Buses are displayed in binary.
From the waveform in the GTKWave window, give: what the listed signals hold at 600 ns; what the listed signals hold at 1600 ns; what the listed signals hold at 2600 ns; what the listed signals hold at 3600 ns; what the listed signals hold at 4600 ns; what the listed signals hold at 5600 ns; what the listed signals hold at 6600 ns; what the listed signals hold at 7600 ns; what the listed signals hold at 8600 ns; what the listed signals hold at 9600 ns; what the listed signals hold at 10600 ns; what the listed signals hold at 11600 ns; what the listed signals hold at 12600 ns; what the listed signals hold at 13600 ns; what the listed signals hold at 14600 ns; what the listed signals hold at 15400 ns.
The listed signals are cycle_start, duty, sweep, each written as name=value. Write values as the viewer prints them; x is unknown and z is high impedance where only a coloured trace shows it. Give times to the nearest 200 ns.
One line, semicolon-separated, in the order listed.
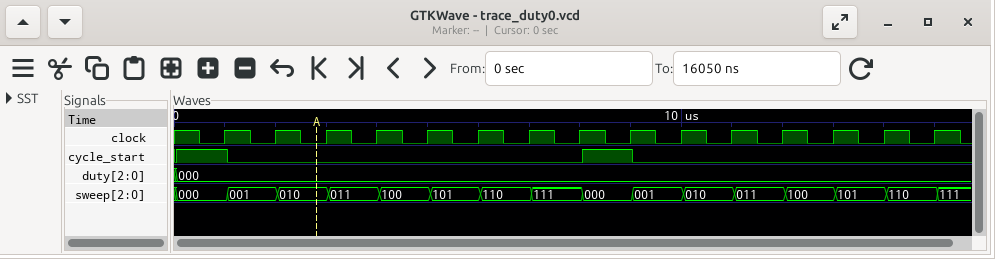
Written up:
cycle_start=1, duty=000, sweep=000; cycle_start=0, duty=000, sweep=001; cycle_start=0, duty=000, sweep=010; cycle_start=0, duty=000, sweep=011; cycle_start=0, duty=000, sweep=100; cycle_start=0, duty=000, sweep=101; cycle_start=0, duty=000, sweep=110; cycle_start=0, duty=000, sweep=111; cycle_start=1, duty=000, sweep=000; cycle_start=0, duty=000, sweep=001; cycle_start=0, duty=000, sweep=010; cycle_start=0, duty=000, sweep=011; cycle_start=0, duty=000, sweep=100; cycle_start=0, duty=000, sweep=101; cycle_start=0, duty=000, sweep=110; cycle_start=0, duty=000, sweep=111
